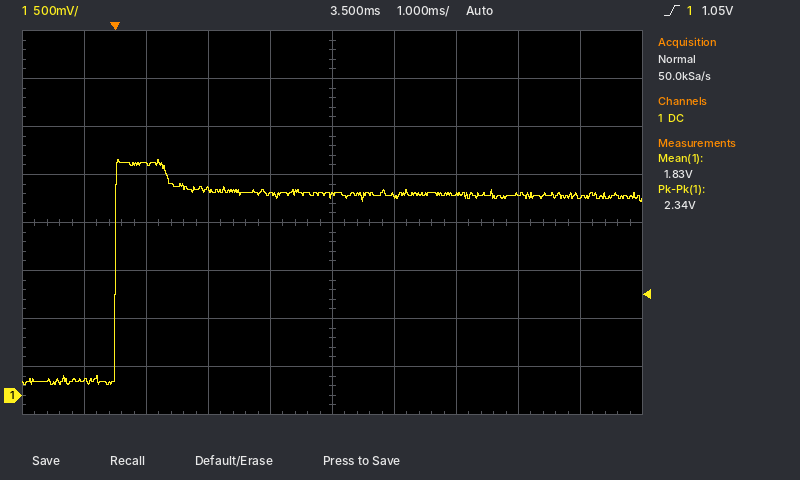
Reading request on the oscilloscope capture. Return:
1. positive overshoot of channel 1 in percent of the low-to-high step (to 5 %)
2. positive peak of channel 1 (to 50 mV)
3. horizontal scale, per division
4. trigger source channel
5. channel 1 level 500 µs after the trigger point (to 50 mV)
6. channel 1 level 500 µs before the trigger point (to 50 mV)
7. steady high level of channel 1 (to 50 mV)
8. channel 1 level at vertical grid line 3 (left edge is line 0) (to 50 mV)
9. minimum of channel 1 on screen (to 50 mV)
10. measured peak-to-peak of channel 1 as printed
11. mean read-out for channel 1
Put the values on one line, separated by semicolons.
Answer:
20 %; 2.45 V; 1 ms; channel 1; 2.40 V; 150 mV; 2.10 V; 2.15 V; 100 mV; 2.34 V; 1.83 V
